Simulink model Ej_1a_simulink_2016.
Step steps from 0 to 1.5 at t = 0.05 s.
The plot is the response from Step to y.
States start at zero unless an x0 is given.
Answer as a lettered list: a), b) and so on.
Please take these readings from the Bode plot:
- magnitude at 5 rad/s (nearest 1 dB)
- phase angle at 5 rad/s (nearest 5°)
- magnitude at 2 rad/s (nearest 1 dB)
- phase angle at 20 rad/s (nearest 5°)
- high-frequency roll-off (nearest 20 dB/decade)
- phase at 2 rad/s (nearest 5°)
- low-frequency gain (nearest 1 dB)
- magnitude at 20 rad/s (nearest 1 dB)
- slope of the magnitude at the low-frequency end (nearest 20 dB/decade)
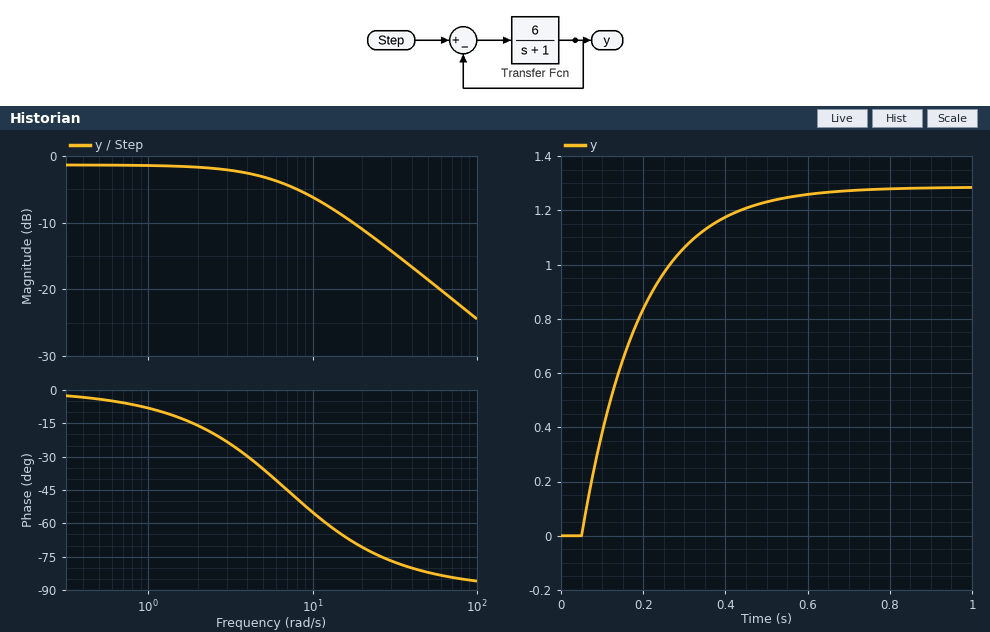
a) -3 dB
b) -35°
c) -2 dB
d) -70°
e) -20 dB/decade
f) -15°
g) -1 dB
h) -11 dB
i) 0 dB/decade
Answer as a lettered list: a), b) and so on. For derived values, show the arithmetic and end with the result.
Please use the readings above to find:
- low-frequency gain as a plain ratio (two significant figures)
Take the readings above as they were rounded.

a) 10^(-1 / 20) = 0.89
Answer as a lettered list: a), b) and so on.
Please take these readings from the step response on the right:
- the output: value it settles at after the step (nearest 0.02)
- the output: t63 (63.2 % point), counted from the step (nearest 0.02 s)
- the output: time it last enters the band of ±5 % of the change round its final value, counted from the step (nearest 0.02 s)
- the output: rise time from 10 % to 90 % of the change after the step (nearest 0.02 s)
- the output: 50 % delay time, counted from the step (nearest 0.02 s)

a) 1.28
b) 0.14 s
c) 0.42 s
d) 0.32 s
e) 0.10 s
